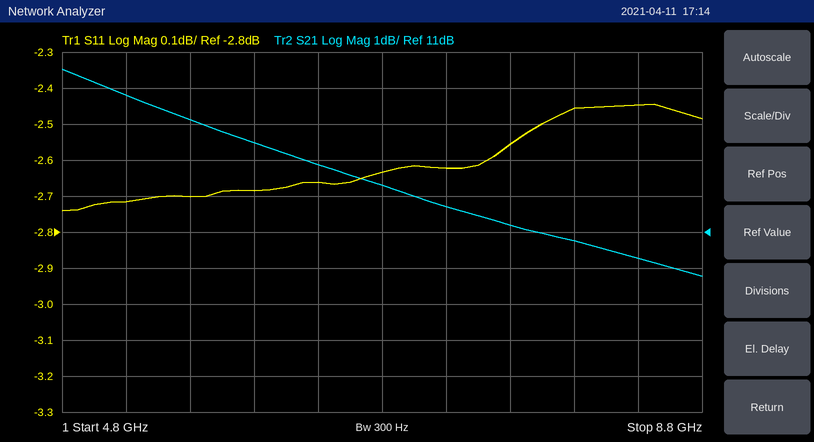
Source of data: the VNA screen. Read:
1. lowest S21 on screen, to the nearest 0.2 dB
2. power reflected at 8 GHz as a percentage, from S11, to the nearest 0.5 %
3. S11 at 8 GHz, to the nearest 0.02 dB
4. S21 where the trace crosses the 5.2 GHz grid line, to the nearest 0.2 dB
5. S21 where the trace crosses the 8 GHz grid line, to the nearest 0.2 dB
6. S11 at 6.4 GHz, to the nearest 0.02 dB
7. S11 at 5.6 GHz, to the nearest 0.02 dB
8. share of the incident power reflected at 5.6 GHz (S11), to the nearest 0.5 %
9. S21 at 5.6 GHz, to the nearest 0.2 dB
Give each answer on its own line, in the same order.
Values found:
9.8 dB
57.0 %
-2.46 dB
14.8 dB
10.8 dB
-2.66 dB
-2.70 dB
53.5 %
14.2 dB
